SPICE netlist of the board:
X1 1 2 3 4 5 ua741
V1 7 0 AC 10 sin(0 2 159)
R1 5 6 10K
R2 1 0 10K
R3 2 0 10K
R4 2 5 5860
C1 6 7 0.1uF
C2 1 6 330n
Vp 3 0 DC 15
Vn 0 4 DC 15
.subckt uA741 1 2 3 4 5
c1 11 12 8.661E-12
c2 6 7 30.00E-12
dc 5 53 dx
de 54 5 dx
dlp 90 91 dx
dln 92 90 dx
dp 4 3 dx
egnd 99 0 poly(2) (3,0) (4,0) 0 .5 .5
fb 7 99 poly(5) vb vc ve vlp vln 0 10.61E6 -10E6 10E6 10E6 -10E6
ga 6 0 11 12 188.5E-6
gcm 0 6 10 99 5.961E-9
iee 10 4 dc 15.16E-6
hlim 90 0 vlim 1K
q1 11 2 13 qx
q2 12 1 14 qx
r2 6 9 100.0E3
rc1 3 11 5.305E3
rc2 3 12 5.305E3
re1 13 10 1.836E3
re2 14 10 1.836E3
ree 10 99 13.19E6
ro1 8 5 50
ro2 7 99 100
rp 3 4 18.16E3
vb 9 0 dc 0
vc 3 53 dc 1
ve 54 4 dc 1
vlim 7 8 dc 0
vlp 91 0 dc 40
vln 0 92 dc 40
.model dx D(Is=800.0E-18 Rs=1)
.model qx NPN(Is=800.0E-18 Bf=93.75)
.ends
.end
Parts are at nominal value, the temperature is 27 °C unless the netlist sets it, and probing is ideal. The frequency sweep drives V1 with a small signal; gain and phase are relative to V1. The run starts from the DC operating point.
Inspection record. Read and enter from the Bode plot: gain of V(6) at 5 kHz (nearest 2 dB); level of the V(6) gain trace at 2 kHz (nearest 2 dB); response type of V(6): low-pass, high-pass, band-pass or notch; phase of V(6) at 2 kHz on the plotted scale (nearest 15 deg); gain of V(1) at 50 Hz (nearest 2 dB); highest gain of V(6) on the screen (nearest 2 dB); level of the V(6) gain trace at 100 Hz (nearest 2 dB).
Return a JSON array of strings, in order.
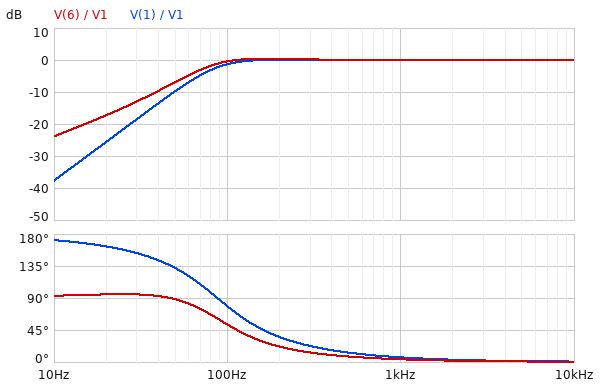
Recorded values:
["0 dB", "0 dB", "high-pass", "0 deg", "-10 dB", "0 dB", "0 dB"]
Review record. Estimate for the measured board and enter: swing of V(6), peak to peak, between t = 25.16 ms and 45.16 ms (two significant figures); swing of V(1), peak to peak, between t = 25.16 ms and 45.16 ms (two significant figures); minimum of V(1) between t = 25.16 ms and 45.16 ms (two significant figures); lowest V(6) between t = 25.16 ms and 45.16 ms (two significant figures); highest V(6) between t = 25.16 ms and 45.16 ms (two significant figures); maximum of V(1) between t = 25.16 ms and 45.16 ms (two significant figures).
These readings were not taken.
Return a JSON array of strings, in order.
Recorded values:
["4.2 V", "4.0 V", "-2.0 V", "-2.1 V", "2.1 V", "2.0 V"]
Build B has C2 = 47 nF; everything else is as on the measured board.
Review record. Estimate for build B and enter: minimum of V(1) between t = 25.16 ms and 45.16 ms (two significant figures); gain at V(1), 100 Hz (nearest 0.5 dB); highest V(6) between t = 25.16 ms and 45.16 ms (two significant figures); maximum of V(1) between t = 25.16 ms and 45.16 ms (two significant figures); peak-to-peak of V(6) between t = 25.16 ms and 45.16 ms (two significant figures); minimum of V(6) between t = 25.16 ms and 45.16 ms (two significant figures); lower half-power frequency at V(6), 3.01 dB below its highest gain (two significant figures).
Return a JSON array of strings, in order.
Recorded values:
["-720 mV", "-15.5 dB", "1.7 V", "720 mV", "3.4 V", "-1.7 V", "140 Hz"]
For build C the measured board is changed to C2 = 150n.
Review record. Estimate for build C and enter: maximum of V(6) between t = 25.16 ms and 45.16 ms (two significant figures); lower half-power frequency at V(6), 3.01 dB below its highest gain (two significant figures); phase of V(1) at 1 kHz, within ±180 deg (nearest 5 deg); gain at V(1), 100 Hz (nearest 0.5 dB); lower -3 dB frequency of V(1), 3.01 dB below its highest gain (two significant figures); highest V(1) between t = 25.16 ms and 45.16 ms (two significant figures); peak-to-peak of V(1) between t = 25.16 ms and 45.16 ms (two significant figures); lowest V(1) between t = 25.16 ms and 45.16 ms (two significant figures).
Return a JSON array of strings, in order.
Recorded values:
["2.1 V", "98 Hz", "10 deg", "-5.5 dB", "120 Hz", "1.8 V", "3.5 V", "-1.8 V"]
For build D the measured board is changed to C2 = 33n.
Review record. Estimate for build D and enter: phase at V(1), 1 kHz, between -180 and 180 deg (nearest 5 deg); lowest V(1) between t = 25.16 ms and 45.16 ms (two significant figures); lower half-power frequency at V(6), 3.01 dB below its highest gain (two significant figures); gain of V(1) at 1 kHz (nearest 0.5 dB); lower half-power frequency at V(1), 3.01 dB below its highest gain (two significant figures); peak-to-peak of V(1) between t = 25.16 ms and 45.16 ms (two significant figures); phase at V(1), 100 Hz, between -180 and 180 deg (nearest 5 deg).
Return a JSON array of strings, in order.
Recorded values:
["30 deg", "-500 mV", "150 Hz", "-0.5 dB", "420 Hz", "1.0 V", "140 deg"]
